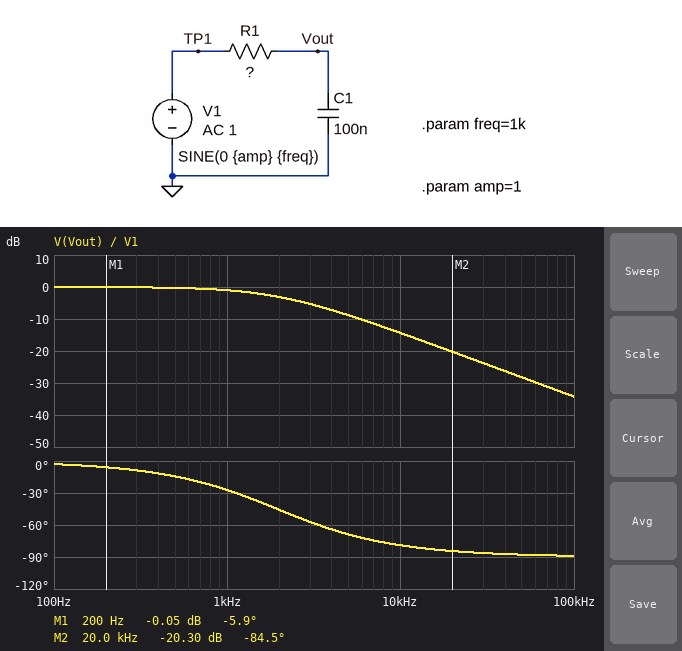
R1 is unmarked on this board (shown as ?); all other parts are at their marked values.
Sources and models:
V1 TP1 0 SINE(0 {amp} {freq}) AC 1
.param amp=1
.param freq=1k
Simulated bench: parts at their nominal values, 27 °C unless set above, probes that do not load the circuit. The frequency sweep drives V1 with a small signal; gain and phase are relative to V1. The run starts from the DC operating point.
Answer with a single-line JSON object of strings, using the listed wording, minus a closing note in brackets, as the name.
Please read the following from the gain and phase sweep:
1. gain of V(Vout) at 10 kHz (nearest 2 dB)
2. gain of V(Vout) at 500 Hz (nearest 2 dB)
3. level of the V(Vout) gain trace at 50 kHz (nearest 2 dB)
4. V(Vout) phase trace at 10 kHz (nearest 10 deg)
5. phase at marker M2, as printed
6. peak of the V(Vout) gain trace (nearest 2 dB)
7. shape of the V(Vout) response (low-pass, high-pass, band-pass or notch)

{"gain of V(Vout) at 10 kHz": "-14 dB", "gain of V(Vout) at 500 Hz": "0 dB", "level of the V(Vout) gain trace at 50 kHz": "-28 dB", "V(Vout) phase trace at 10 kHz": "-80 deg", "phase at marker M2, as printed": "-84.5 deg", "peak of the V(Vout) gain trace": "0 dB", "shape of the V(Vout) response": "low-pass"}
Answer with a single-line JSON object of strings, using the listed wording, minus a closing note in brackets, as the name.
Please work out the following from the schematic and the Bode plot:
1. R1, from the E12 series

{"R1, from the E12 series": "820 Ω"}
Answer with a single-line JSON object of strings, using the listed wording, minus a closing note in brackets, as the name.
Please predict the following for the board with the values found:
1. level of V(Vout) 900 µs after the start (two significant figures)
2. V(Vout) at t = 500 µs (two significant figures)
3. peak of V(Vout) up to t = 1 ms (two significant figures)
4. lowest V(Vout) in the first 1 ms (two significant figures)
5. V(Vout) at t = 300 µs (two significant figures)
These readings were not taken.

{"level of V(Vout) 900 µs after the start": "-790 mV", "V(Vout) at t = 500 µs": "410 mV", "peak of V(Vout) up to t = 1 ms": "900 mV", "lowest V(Vout) in the first 1 ms": "-890 mV", "V(Vout) at t = 300 µs": "890 mV"}
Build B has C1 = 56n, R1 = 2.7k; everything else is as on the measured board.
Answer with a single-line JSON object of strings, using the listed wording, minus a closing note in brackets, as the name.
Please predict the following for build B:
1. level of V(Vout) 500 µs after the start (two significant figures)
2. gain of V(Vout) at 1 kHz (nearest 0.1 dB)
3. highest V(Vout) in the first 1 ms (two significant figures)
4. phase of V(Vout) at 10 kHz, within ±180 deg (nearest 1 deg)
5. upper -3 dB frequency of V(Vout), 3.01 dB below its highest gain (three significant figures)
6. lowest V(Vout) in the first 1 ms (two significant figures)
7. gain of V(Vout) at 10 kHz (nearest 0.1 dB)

{"level of V(Vout) 500 µs after the start": "520 mV", "gain of V(Vout) at 1 kHz": "-2.8 dB", "highest V(Vout) in the first 1 ms": "770 mV", "phase of V(Vout) at 10 kHz, within ±180 deg": "-84 deg", "upper -3 dB frequency of V(Vout), 3.01 dB below its highest gain": "1.05 kHz", "lowest V(Vout) in the first 1 ms": "-720 mV", "gain of V(Vout) at 10 kHz": "-19.6 dB"}
